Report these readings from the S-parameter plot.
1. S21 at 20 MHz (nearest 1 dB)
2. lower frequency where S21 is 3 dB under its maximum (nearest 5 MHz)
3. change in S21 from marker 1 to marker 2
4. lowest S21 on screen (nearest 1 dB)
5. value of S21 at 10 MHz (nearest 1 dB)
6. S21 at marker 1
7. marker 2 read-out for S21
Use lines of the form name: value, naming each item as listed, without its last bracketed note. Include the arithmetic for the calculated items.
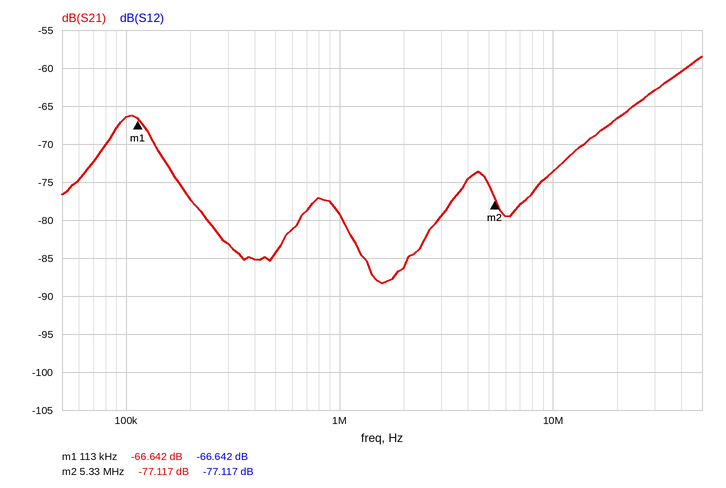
S21 at 20 MHz: -67 dB
lower frequency where S21 is 3 dB under its maximum: 35 MHz
change in S21 from marker 1 to marker 2: -77.117 − (-66.642) = -10.475 dB
lowest S21 on screen: -88 dB
value of S21 at 10 MHz: -74 dB
S21 at marker 1: -66.642 dB
marker 2 read-out for S21: -77.117 dB
